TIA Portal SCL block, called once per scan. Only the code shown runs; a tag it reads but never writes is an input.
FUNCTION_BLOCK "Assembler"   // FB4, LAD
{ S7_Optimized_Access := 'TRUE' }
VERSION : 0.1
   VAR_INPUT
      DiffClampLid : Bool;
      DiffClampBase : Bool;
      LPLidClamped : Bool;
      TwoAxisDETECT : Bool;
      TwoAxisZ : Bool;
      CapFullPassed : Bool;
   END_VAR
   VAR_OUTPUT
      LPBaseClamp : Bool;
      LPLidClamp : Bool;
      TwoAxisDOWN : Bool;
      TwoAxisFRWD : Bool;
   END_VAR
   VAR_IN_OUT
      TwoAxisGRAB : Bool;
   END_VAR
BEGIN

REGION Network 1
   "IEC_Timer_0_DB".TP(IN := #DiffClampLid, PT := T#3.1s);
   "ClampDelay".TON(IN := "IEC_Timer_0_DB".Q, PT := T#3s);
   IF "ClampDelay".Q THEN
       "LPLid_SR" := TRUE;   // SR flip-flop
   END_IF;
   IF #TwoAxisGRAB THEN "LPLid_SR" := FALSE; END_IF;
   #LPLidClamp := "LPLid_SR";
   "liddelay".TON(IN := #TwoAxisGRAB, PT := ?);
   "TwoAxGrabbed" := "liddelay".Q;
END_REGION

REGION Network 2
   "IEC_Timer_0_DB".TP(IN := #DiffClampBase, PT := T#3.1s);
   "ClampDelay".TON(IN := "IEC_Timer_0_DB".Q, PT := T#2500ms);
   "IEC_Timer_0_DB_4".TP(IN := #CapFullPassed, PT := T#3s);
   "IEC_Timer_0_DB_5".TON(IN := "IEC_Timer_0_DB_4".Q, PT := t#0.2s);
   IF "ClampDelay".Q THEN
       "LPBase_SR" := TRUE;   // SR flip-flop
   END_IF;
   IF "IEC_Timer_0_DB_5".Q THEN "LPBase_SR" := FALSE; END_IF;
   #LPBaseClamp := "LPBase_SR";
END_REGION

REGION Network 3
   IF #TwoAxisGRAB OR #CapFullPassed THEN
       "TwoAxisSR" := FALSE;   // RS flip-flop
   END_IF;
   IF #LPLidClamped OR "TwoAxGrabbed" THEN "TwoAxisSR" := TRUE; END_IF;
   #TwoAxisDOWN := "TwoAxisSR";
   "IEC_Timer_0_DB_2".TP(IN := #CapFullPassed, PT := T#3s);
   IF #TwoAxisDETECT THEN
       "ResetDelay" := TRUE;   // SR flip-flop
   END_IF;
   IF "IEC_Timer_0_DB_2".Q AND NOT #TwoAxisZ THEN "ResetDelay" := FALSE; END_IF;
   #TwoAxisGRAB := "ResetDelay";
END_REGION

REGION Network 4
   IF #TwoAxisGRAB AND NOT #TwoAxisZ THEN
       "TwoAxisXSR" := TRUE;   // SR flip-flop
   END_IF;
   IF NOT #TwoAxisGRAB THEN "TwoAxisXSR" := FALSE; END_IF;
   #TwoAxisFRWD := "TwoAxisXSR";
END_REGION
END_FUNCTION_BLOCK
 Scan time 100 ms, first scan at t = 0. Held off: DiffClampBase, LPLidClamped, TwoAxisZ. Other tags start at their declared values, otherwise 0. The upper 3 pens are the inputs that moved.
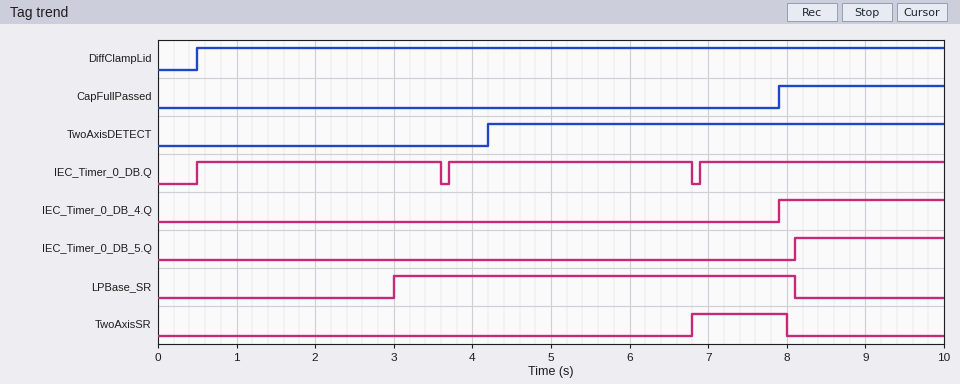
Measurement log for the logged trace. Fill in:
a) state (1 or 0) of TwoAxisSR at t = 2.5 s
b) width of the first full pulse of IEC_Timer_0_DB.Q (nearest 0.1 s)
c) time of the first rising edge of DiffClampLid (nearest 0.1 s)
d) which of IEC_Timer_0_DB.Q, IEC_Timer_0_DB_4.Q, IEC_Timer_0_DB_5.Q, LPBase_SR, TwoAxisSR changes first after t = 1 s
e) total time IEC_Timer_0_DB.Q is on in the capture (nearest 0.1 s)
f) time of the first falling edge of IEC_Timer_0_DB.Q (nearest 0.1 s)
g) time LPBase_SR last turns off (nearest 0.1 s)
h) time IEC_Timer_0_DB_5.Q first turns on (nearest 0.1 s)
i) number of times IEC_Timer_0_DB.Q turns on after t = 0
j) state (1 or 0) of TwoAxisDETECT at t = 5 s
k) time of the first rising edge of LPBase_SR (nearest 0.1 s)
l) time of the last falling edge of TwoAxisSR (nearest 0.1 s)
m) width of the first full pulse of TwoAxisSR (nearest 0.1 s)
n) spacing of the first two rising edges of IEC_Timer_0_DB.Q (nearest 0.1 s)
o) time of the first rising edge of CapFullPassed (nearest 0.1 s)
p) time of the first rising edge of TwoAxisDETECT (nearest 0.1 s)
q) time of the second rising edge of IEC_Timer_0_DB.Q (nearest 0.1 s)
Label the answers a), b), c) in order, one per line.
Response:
a) 0
b) 3.1 s
c) 0.5 s
d) LPBase_SR
e) 9.3 s
f) 3.6 s
g) 8.1 s
h) 8.1 s
i) 3
j) 1
k) 3.0 s
l) 8.0 s
m) 1.2 s
n) 3.2 s
o) 7.9 s
p) 4.2 s
q) 3.7 s
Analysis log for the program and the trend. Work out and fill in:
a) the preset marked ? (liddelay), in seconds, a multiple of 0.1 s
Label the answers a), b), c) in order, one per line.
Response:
a) 2.5 s
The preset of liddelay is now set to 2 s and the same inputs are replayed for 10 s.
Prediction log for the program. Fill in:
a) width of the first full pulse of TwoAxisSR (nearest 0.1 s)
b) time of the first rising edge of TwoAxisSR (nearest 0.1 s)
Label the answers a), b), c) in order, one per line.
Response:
a) 1.7 s
b) 6.3 s
